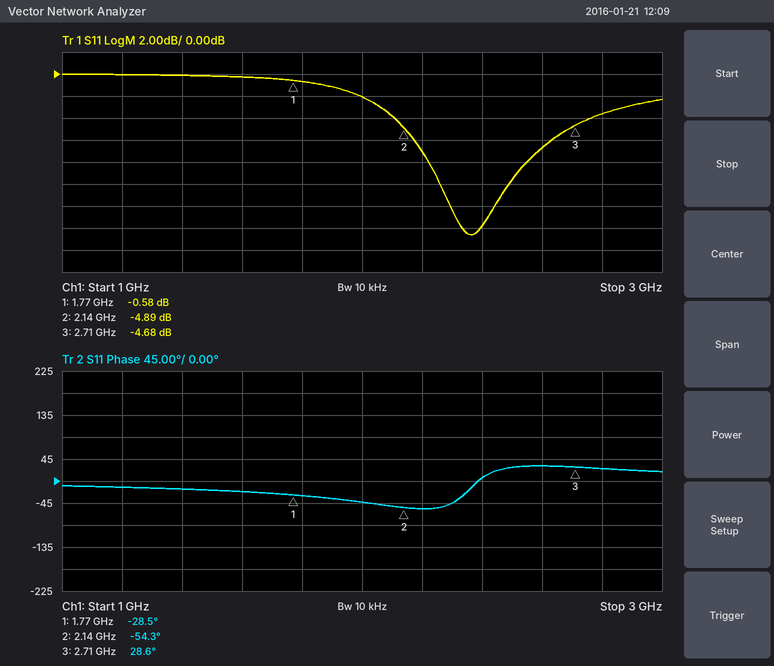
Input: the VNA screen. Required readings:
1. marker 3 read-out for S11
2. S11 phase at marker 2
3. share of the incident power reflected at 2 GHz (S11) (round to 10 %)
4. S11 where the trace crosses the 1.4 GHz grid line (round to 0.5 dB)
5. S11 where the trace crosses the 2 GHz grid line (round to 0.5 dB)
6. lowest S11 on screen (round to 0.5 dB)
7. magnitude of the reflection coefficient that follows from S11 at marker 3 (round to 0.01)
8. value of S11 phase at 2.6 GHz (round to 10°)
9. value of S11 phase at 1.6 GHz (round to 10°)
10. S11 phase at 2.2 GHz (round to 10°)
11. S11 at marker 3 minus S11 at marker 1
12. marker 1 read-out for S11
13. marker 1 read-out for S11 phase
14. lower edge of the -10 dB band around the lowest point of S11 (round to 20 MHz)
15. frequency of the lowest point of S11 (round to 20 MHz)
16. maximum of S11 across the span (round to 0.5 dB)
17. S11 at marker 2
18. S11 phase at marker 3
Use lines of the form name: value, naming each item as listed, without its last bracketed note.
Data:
marker 3 read-out for S11: -4.68 dB
S11 phase at marker 2: -54.3°
share of the incident power reflected at 2 GHz (S11): 60 %
S11 where the trace crosses the 1.4 GHz grid line: 0.0 dB
S11 where the trace crosses the 2 GHz grid line: -2.0 dB
lowest S11 on screen: -14.5 dB
magnitude of the reflection coefficient that follows from S11 at marker 3: 0.58
value of S11 phase at 2.6 GHz: 30°
value of S11 phase at 1.6 GHz: -20°
S11 phase at 2.2 GHz: -60°
S11 at marker 3 minus S11 at marker 1: -4.10 dB
marker 1 read-out for S11: -0.58 dB
marker 1 read-out for S11 phase: -28.5°
lower edge of the -10 dB band around the lowest point of S11: 2.26 GHz
frequency of the lowest point of S11: 2.36 GHz
maximum of S11 across the span: 0.0 dB
S11 at marker 2: -4.89 dB
S11 phase at marker 3: 28.6°
